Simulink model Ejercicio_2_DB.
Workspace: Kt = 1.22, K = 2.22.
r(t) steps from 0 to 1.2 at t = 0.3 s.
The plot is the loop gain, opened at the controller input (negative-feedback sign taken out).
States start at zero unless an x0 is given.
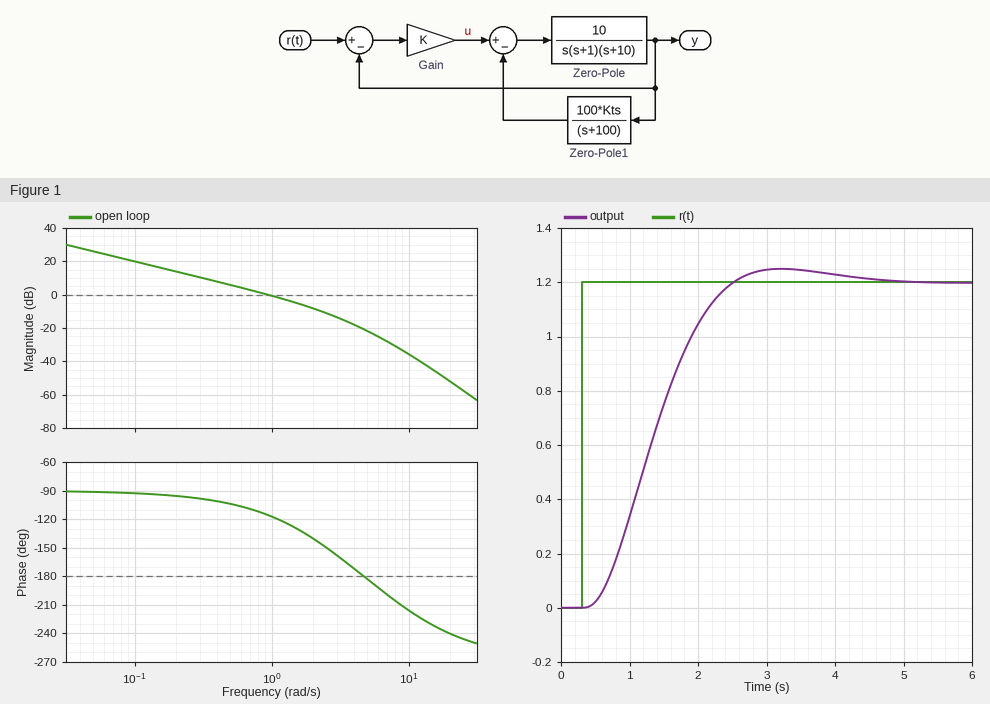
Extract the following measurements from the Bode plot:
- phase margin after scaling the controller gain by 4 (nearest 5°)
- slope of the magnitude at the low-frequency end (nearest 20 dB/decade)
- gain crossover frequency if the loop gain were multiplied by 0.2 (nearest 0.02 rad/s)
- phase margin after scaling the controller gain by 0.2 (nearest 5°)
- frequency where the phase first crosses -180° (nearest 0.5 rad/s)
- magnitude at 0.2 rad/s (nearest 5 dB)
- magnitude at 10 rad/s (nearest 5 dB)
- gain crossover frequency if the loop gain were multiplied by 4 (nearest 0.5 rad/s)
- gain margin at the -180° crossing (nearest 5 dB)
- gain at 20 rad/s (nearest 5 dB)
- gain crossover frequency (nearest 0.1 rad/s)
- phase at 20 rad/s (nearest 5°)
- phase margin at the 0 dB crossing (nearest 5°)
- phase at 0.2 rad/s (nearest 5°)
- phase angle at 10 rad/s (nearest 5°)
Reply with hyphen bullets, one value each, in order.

- 25°
- -20 dB/decade
- 0.20 rad/s
- 85°
- 4.5 rad/s
- 15 dB
- -35 dB
- 2.5 rad/s
- 20 dB
- -50 dB
- 0.9 rad/s
- -240°
- 65°
- -95°
- -215°
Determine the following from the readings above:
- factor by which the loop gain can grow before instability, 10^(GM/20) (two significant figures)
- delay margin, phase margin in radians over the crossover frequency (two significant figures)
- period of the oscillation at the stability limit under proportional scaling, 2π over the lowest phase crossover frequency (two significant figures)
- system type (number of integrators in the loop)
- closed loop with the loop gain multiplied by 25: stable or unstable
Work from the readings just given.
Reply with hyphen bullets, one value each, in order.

- 10
- 1.3 s
- 1.4 s
- 1
- unstable
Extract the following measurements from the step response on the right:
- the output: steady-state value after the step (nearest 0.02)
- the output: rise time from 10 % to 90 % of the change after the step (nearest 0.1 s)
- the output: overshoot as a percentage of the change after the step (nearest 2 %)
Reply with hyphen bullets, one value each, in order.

- 1.20
- 1.4 s
- 4 %
